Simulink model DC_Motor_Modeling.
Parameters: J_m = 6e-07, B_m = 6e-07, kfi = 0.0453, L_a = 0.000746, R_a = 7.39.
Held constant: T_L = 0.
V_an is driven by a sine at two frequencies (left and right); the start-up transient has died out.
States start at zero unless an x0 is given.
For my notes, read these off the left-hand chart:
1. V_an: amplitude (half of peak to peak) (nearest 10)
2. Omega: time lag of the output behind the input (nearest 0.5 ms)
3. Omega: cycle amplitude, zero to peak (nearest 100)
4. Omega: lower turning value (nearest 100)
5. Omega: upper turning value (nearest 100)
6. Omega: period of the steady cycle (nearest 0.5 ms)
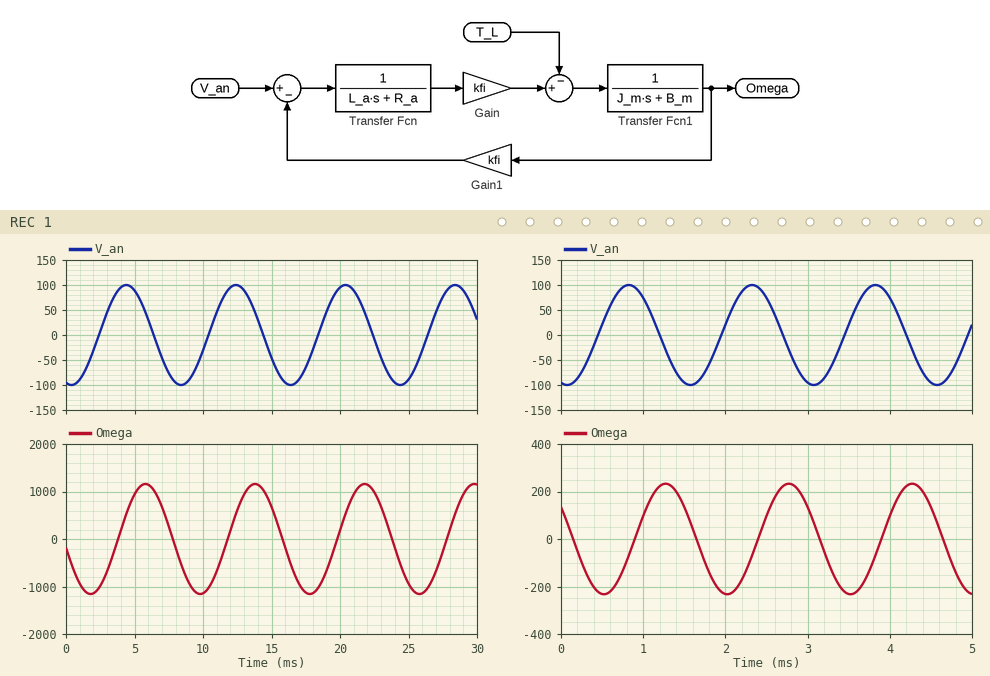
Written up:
100
1.5 ms
1200
-1200
1200
8.0 ms
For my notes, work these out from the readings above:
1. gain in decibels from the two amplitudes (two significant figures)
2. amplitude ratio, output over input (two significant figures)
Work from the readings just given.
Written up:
22 dB
12
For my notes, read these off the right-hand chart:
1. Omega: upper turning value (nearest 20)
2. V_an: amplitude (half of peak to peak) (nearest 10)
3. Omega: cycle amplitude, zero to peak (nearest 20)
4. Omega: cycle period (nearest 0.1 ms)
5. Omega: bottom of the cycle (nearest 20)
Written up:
240
100
240
1.5 ms
-240
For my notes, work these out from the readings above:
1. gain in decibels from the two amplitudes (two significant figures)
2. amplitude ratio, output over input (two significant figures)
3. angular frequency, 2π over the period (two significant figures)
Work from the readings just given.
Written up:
7.6 dB
2.4
4.2 rad/ms
